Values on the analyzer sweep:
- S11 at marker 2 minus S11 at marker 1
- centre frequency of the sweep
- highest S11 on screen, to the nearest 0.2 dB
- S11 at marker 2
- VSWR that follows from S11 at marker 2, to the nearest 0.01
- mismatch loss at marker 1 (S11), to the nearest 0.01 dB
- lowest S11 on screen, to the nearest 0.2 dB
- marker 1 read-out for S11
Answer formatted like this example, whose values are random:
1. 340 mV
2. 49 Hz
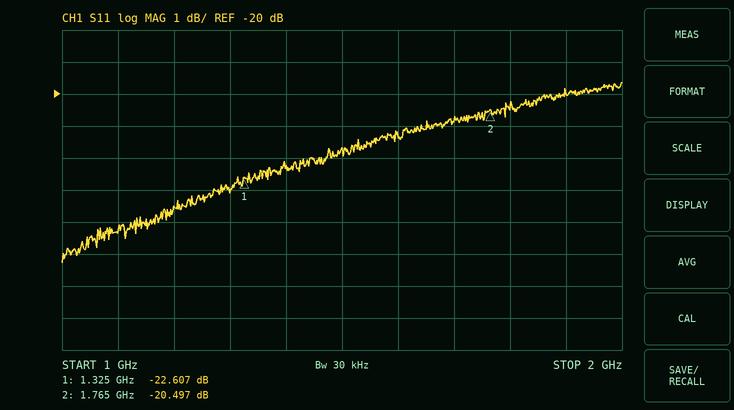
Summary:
1. 2.110 dB
2. 1.5 GHz
3. -19.6 dB
4. -20.497 dB
5. 1.21
6. 0.02 dB
7. -25.2 dB
8. -22.607 dB
